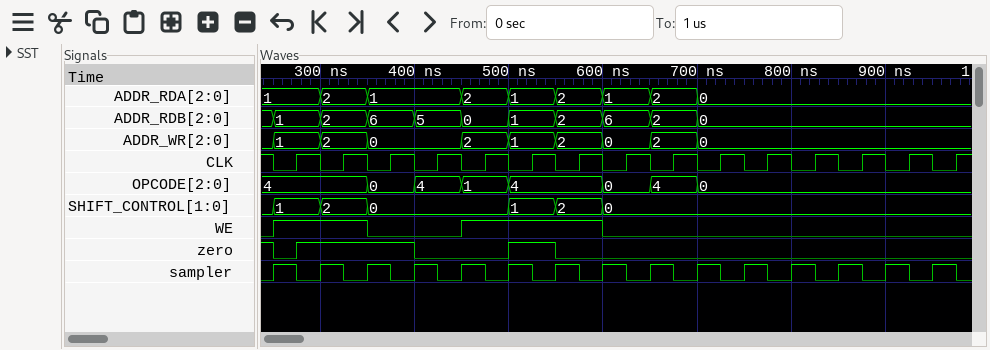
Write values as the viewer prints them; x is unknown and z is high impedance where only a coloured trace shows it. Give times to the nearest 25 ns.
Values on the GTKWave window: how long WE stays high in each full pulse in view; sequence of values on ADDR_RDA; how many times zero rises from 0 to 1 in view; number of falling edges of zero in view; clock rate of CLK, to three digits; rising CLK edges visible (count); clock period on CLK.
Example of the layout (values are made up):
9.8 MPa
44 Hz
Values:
100 ns, 150 ns
1, 2, 1, 2, 1, 2, 1, 2, 0
2
3
20.0 MHz
15
50 ns
